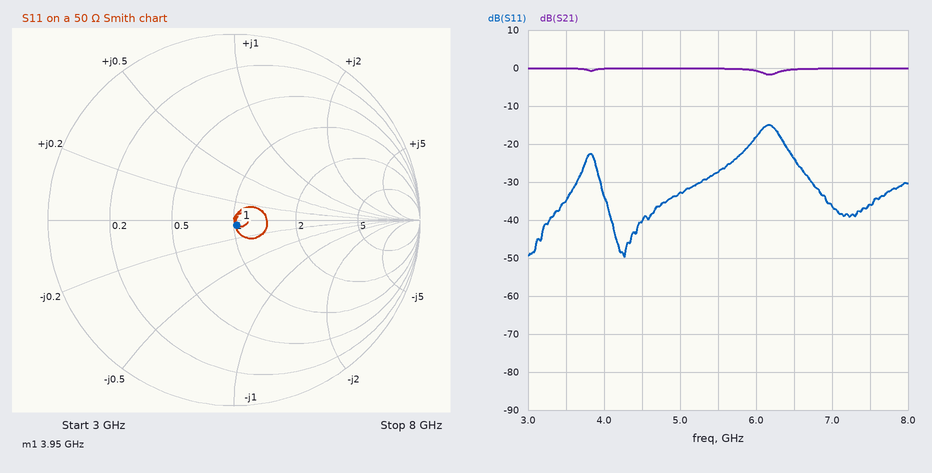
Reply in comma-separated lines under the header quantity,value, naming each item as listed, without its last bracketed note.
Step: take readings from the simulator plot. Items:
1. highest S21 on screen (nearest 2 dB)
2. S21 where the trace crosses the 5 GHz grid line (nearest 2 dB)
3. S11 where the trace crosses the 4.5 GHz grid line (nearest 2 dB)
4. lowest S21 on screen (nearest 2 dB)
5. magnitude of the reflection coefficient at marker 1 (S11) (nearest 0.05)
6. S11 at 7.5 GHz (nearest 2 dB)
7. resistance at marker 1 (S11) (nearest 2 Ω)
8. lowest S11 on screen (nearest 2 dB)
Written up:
quantity,value
highest S21 on screen,0 dB
S21 where the trace crosses the 5 GHz grid line,0 dB
S11 where the trace crosses the 4.5 GHz grid line,-40 dB
lowest S21 on screen,-2 dB
magnitude of the reflection coefficient at marker 1 (S11),0.05
S11 at 7.5 GHz,-36 dB
resistance at marker 1 (S11),52 Ω
lowest S11 on screen,-50 dB
